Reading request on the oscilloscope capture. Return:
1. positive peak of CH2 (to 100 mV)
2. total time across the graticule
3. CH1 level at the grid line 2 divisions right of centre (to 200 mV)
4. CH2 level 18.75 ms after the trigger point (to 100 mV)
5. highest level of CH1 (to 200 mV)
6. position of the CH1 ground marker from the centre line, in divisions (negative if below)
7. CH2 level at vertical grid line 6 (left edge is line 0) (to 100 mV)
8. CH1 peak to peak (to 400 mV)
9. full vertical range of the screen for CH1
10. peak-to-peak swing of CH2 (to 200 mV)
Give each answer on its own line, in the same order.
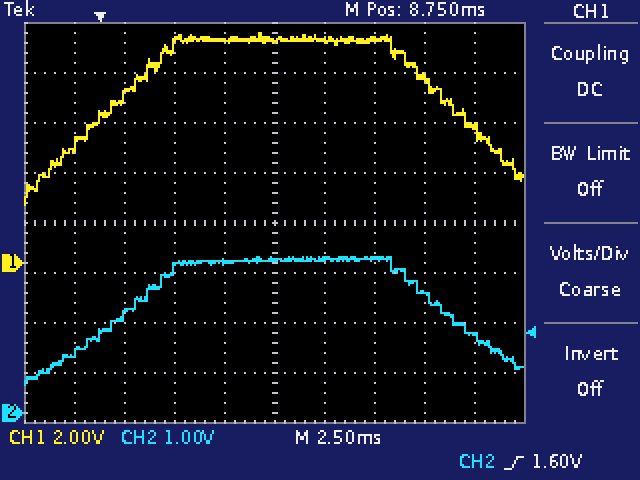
3.1 V
25 ms
9.0 V
1.5 V
9.2 V
-0.8 div
3.1 V
6.8 V
16 V
2.6 V
